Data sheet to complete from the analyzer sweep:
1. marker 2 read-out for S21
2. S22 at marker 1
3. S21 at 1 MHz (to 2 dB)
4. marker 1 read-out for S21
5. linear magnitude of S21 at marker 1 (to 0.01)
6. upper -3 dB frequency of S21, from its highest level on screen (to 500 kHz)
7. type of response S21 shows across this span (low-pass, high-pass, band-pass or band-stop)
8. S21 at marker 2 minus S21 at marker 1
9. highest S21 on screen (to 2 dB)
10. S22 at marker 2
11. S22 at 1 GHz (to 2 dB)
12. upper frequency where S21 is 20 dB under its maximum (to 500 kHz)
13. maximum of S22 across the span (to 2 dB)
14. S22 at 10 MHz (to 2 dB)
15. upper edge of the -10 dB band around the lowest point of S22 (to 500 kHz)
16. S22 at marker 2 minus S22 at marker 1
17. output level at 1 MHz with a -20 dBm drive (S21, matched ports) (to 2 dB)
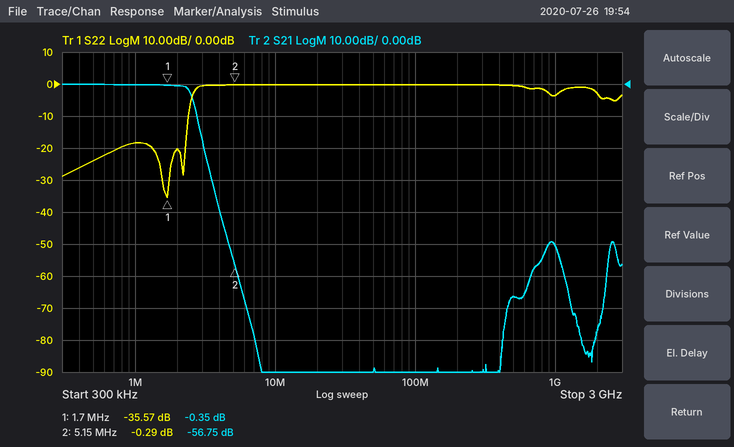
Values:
-56.75 dB
-35.57 dB
0 dB
-0.35 dB
0.96
2.5 MHz
low-pass
-56.40 dB
0 dB
-0.29 dB
-4 dB
3.0 MHz
0 dB
0 dB
2.5 MHz
35.28 dB
-20 dBm
